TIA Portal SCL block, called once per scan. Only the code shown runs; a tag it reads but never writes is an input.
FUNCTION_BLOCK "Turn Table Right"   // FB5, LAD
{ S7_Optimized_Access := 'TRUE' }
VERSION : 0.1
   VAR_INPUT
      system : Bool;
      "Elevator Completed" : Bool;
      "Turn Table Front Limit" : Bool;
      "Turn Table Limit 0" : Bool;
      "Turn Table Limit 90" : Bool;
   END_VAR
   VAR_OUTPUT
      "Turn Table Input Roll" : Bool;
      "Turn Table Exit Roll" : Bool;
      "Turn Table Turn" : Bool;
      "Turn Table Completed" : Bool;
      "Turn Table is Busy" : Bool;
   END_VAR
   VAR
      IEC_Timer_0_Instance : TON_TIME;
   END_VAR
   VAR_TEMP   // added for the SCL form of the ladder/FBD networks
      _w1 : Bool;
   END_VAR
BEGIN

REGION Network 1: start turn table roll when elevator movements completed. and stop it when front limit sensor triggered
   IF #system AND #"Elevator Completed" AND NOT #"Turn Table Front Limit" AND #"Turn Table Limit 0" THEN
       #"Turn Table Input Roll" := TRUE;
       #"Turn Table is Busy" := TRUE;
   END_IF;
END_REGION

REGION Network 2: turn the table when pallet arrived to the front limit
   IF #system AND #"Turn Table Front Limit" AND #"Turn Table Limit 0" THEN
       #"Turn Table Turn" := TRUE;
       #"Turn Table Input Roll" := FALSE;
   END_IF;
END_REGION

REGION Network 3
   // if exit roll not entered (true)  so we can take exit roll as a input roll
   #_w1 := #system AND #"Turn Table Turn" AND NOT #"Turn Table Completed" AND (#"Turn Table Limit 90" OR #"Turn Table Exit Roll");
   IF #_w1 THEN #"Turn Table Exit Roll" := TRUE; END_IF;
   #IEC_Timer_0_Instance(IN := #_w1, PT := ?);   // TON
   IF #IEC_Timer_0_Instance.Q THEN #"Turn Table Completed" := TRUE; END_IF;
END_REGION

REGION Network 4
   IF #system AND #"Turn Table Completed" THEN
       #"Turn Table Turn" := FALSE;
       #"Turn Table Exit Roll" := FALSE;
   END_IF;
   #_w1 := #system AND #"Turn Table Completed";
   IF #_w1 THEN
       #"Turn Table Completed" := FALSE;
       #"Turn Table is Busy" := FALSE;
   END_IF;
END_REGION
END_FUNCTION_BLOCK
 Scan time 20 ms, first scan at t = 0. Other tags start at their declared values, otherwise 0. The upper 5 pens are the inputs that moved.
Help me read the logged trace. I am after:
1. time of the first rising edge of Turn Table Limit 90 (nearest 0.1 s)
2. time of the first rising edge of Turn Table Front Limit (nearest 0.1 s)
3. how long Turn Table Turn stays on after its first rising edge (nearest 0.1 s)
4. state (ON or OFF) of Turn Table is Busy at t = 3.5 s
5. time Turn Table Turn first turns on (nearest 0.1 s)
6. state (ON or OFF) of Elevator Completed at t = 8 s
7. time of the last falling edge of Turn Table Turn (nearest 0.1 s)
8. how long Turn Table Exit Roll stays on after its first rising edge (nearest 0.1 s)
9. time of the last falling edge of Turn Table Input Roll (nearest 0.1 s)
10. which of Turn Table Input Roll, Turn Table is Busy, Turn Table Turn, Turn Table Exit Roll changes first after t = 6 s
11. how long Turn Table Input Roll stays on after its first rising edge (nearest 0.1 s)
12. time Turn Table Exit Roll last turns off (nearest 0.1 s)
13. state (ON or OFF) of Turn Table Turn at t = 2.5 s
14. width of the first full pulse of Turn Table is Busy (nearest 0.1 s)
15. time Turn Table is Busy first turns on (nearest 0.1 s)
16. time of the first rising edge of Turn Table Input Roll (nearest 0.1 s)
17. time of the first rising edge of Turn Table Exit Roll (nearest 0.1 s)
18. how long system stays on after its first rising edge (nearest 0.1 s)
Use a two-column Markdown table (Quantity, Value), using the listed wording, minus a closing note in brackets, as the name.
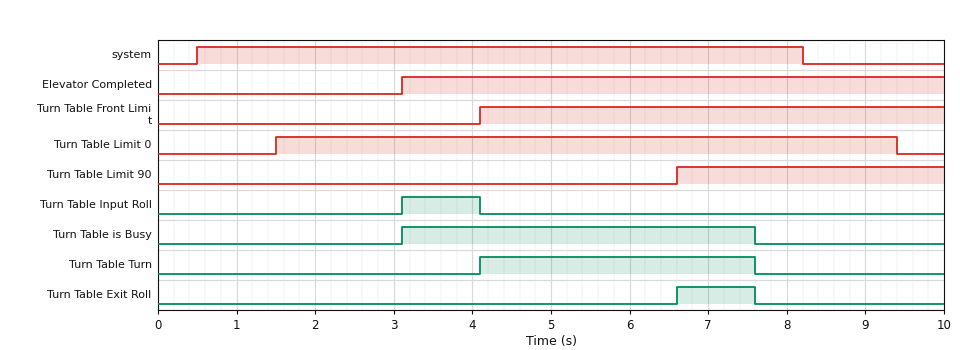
| Quantity | Value |
|---|---|
| time of the first rising edge of Turn Table Limit 90 | 6.6 s |
| time of the first rising edge of Turn Table Front Limit | 4.1 s |
| how long Turn Table Turn stays on after its first rising edge | 3.5 s |
| state (ON or OFF) of Turn Table is Busy at t = 3.5 s | ON |
| time Turn Table Turn first turns on | 4.1 s |
| state (ON or OFF) of Elevator Completed at t = 8 s | ON |
| time of the last falling edge of Turn Table Turn | 7.6 s |
| how long Turn Table Exit Roll stays on after its first rising edge | 1.0 s |
| time of the last falling edge of Turn Table Input Roll | 4.1 s |
| which of Turn Table Input Roll, Turn Table is Busy, Turn Table Turn, Turn Table Exit Roll changes first after t = 6 s | Turn Table Exit Roll |
| how long Turn Table Input Roll stays on after its first rising edge | 1.0 s |
| time Turn Table Exit Roll last turns off | 7.6 s |
| state (ON or OFF) of Turn Table Turn at t = 2.5 s | OFF |
| width of the first full pulse of Turn Table is Busy | 4.5 s |
| time Turn Table is Busy first turns on | 3.1 s |
| time of the first rising edge of Turn Table Input Roll | 3.1 s |
| time of the first rising edge of Turn Table Exit Roll | 6.6 s |
| how long system stays on after its first rising edge | 7.7 s |
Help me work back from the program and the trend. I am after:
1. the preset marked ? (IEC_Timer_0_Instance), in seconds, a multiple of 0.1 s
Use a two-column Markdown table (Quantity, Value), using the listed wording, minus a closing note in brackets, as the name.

| Quantity | Value |
|---|---|
| the preset marked ? (IEC_Timer_0_Instance), in seconds, a multiple of 0.1 s | 1.0 s |
